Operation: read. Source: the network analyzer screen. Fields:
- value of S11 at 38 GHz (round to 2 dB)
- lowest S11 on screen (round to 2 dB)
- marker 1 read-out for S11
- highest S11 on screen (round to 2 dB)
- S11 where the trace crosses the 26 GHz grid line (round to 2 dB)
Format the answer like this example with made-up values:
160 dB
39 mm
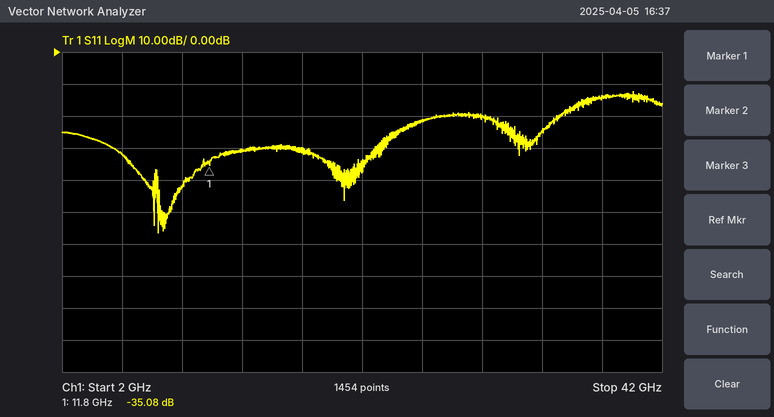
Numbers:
-14 dB
-56 dB
-35.08 dB
-12 dB
-22 dB
